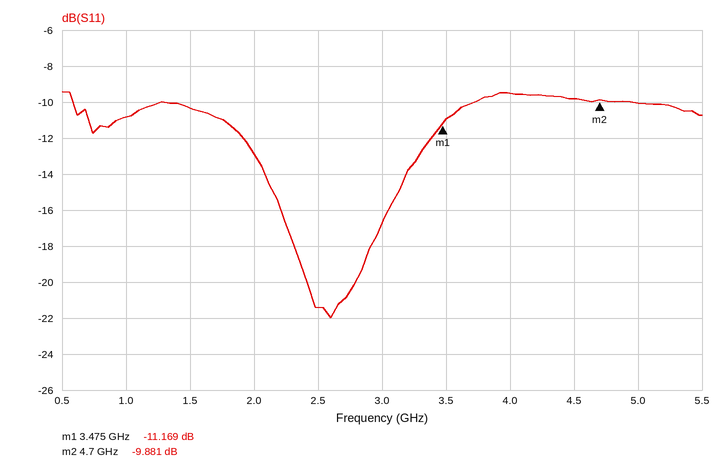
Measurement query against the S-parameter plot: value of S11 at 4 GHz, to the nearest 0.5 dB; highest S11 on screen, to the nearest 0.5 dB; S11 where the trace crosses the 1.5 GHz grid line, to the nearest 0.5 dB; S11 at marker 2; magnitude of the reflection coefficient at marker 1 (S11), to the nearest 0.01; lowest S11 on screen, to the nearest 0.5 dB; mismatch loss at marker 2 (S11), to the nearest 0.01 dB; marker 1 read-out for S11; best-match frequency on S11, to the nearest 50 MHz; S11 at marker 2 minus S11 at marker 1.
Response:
-9.5 dB
-9.5 dB
-10.5 dB
-9.881 dB
0.28
-22.0 dB
0.47 dB
-11.169 dB
2.60 GHz
1.288 dB
